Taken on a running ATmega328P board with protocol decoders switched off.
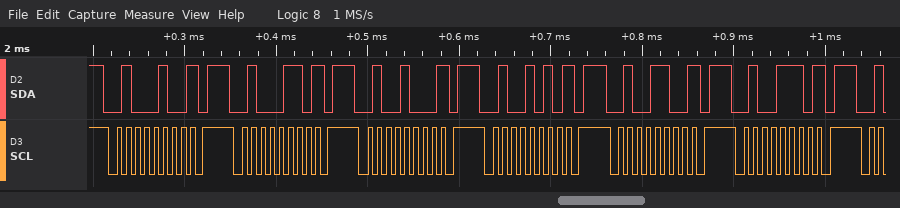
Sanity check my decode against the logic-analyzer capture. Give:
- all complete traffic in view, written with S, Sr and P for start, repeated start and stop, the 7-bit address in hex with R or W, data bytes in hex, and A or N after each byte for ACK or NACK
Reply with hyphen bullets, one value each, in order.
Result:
- S 22W N P S 23W N P S 24W N P S 25W N P S 26W N P S 27W N P
